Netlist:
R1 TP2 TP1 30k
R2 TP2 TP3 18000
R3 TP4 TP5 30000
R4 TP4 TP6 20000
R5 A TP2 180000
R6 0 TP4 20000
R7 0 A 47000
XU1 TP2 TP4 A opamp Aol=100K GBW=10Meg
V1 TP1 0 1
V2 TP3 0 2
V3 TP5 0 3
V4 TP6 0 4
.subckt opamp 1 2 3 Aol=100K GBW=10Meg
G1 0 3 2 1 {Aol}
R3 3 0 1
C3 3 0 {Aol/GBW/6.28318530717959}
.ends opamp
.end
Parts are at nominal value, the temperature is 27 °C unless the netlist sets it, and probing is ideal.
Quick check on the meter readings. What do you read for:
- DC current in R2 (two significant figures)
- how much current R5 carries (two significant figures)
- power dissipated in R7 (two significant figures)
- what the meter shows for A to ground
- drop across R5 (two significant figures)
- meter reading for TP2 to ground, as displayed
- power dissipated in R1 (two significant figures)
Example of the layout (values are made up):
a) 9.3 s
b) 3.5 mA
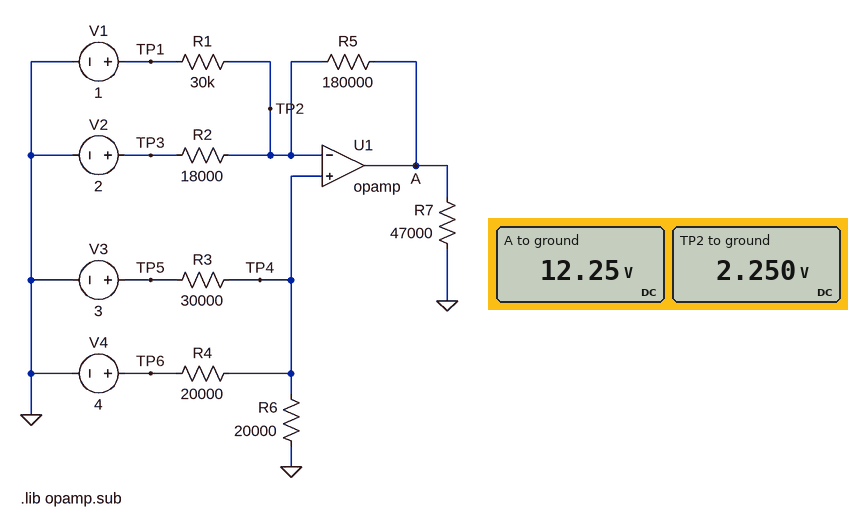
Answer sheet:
a) 14 µA
b) 56 µA
c) 3.2 mW
d) 12.25 V
e) 10 V
f) 2.250 V
g) 52 µW
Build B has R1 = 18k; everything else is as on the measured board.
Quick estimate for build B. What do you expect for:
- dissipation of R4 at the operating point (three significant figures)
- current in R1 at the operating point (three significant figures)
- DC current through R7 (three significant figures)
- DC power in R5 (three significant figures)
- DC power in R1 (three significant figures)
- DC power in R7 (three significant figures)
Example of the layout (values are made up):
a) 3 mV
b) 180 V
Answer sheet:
a) 153 µW
b) 69.4 µA
c) 367 µA
d) 1.25 mW
e) 86.8 µW
f) 6.33 mW
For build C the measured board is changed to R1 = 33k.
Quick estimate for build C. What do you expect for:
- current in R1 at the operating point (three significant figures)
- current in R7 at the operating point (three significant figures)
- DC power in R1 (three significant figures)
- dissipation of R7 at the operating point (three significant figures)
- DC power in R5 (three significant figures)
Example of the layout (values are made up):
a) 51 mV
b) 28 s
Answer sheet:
a) 37.9 µA
b) 246 µA
c) 47.3 µW
d) 2.85 mW
e) 482 µW
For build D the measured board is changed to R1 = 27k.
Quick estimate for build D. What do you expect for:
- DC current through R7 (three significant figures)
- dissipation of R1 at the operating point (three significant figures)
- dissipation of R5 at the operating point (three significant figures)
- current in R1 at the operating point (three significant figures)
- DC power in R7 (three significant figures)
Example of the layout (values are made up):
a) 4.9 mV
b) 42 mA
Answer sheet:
a) 278 µA
b) 57.9 µW
c) 652 µW
d) 46.3 µA
e) 3.64 mW
